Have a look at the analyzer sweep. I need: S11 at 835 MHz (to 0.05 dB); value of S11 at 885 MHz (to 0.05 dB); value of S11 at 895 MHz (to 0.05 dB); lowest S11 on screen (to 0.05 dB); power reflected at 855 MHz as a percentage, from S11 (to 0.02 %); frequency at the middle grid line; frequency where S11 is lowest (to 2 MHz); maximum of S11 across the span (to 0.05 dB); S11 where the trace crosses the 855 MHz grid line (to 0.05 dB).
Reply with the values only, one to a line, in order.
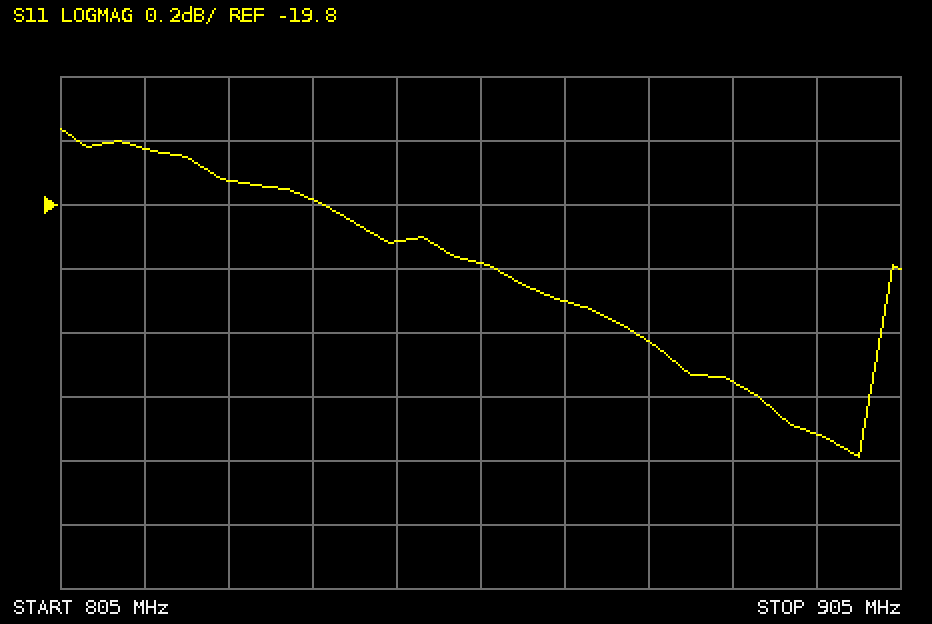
-19.80 dB
-20.35 dB
-20.50 dB
-20.60 dB
1.00 %
855 MHz
900 MHz
-19.55 dB
-20.00 dB
